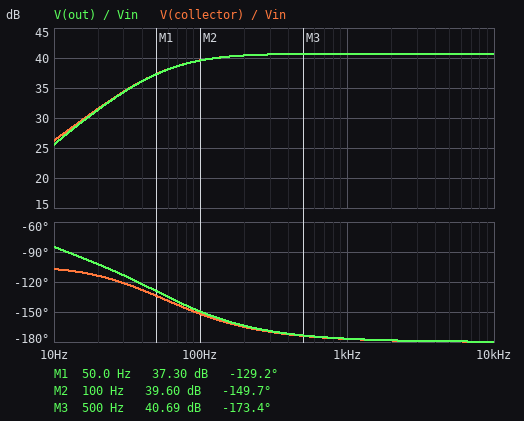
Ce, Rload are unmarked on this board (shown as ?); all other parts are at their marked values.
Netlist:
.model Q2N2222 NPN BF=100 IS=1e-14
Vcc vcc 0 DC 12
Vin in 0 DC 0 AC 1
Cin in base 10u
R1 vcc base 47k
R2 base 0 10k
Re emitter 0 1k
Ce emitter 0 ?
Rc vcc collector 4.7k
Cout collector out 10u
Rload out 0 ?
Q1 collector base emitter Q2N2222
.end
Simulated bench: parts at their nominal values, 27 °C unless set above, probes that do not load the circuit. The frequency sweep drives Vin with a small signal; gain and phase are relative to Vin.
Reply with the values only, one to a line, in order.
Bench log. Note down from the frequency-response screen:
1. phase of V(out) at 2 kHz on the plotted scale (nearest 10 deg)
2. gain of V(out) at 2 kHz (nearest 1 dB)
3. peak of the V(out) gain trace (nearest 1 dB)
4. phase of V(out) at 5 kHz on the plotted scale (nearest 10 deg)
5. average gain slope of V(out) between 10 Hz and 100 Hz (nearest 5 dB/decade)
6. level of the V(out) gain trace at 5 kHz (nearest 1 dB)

-180 deg
41 dB
41 dB
-180 deg
15 dB/decade
41 dB
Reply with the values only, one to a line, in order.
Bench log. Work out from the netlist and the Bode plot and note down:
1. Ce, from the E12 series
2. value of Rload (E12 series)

180 µF
3.9 kΩ
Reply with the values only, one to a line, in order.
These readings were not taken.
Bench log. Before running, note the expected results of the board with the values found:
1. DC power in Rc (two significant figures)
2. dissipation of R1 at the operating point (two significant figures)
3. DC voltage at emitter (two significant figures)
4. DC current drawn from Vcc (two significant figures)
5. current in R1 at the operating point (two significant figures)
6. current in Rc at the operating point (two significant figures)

8.2 mW
2.1 mW
1.3 V
1.5 mA
210 µA
1.3 mA
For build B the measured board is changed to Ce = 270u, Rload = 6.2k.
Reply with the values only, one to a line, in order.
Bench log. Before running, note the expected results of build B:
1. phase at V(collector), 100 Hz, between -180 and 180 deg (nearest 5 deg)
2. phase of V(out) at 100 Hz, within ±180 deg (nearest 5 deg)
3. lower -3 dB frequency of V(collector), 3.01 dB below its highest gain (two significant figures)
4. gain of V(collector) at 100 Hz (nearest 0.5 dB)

-160 deg
-155 deg
39 Hz
42.0 dB
